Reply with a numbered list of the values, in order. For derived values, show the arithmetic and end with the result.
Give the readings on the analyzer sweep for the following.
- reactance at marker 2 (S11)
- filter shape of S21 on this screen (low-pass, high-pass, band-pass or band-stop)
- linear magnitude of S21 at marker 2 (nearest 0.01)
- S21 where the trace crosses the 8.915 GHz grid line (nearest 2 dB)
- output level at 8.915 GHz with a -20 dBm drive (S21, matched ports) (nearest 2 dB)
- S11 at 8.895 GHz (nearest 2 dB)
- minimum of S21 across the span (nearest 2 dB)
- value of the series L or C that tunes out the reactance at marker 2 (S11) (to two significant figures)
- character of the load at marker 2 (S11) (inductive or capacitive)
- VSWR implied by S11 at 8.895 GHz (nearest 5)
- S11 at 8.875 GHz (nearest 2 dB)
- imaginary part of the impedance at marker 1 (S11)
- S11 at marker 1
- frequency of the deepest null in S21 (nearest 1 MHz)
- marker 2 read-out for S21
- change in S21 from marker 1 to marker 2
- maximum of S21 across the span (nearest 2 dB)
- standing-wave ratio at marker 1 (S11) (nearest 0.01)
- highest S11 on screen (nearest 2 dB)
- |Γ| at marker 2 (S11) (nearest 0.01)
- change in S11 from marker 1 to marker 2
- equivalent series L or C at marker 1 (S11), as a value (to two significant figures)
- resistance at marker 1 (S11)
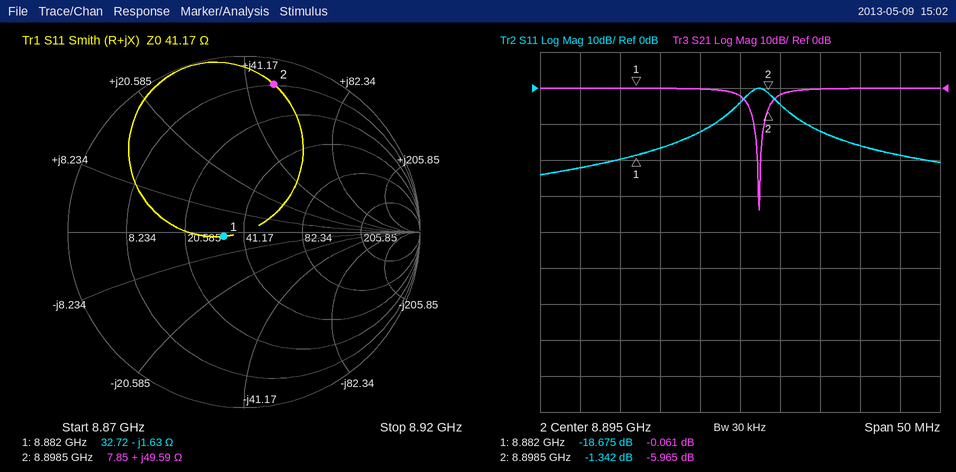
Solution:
1. +49.59 Ω
2. band-stop
3. 10^(-5.965/20) ≈ 0.50
4. 0 dB
5. -20 dBm + (0 dB) = -20 dBm
6. -4 dB
7. -34 dB
8. C = 1/(2π × 8.8985 GHz × 49.59 Ω) ≈ 361 fF, so 360 fF to two significant figures
9. inductive
10. |Γ| = 10^(-4/20) = 0.6310; VSWR = (1 + 0.6310)/(1 − 0.6310) ≈ 4.42, so 5 to the nearest 5
11. -22 dB
12. -1.63 Ω
13. -18.675 dB
14. 8.897 GHz
15. -5.965 dB
16. -5.965 − (-0.061) = -5.904 dB
17. 0 dB
18. 1.26
19. 0 dB
20. 0.86
21. -1.342 − (-18.675) = 17.333 dB
22. C = 1/(2π × 8.882 GHz × 1.63 Ω) ≈ 11 pF
23. 32.72 Ω
